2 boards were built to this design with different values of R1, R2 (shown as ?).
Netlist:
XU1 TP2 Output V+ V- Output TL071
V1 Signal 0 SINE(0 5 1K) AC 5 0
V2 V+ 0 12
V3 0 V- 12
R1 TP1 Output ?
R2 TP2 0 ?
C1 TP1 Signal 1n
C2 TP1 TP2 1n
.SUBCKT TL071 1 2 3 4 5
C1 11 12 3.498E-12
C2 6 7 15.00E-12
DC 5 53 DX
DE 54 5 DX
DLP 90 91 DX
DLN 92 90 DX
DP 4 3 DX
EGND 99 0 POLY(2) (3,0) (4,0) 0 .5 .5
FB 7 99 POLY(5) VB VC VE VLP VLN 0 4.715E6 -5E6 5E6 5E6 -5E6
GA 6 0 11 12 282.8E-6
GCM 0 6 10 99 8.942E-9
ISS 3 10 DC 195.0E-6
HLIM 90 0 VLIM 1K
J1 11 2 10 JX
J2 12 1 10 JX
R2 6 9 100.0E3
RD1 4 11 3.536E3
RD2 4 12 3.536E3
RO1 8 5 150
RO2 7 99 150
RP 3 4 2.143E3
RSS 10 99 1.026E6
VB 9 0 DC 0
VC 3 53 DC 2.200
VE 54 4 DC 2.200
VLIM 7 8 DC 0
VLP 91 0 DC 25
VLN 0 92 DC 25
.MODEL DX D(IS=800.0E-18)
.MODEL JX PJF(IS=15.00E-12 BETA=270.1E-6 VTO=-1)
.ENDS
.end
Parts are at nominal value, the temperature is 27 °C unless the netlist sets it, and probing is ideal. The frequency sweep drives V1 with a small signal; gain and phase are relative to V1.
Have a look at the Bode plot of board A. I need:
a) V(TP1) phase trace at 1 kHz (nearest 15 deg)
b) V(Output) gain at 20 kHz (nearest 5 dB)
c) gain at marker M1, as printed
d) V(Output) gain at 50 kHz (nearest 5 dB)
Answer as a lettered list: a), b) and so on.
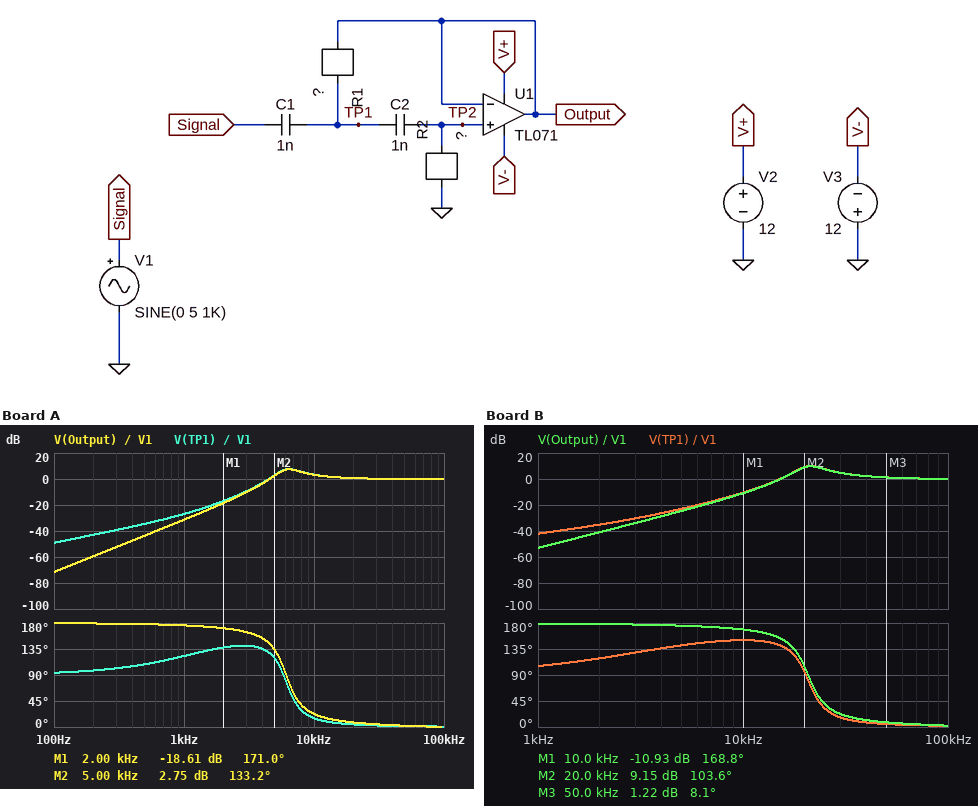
a) 120 deg
b) 0 dB
c) -18.61 dB
d) 0 dB
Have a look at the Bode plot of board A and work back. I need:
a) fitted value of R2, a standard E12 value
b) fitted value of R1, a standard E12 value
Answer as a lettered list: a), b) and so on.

a) 120 kΩ
b) 5.6 kΩ
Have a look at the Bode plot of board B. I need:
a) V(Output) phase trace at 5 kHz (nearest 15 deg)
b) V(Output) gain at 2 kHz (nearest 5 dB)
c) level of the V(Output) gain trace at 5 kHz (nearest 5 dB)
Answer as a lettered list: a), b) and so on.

a) 180 deg
b) -40 dB
c) -25 dB
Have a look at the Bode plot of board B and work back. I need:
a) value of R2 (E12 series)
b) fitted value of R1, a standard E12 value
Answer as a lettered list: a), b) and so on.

a) 47 kΩ
b) 1.2 kΩ
